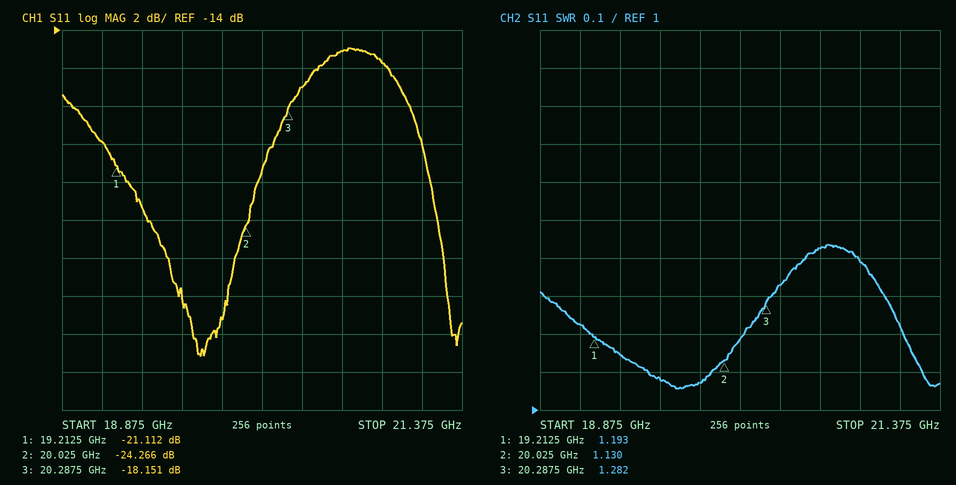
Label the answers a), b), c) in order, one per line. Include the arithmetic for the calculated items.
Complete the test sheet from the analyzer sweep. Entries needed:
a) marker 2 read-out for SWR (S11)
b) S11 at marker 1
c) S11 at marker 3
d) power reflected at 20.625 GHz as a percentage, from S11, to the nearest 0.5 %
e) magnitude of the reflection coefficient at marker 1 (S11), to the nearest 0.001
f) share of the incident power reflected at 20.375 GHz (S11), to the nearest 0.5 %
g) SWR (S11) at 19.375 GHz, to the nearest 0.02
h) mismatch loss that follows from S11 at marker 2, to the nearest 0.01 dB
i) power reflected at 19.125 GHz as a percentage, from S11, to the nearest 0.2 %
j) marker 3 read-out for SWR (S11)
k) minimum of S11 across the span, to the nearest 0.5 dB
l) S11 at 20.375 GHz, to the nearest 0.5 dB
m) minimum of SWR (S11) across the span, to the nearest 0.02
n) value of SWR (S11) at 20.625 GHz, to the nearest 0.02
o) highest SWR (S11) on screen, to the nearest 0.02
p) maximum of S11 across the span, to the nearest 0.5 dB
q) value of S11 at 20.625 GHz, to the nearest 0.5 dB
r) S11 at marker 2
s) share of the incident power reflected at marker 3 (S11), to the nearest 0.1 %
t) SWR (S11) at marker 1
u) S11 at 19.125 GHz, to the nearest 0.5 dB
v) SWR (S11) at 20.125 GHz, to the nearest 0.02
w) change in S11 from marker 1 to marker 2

a) 1.130
b) -21.112 dB
c) -18.151 dB
d) 10^(-15/10) ≈ 3.16 %, so 3.0 % to the nearest 0.5 %
e) 10^(-21.112/20) ≈ 0.088
f) 10^(-17/10) ≈ 2.0 %
g) 1.14
h) −10 log10(1 − 10^(-24.266/10)) ≈ 0.02 dB
i) 10^(-20/10) ≈ 1.0 %
j) 1.282
k) -31.0 dB
l) -17.0 dB
m) 1.06
n) 1.42
o) 1.44
p) -15.0 dB
q) -15.0 dB
r) -24.266 dB
s) 10^(-18.151/10) ≈ 1.5 %
t) 1.193
u) -20.0 dB
v) 1.18
w) -24.266 − (-21.112) = -3.154 dB
